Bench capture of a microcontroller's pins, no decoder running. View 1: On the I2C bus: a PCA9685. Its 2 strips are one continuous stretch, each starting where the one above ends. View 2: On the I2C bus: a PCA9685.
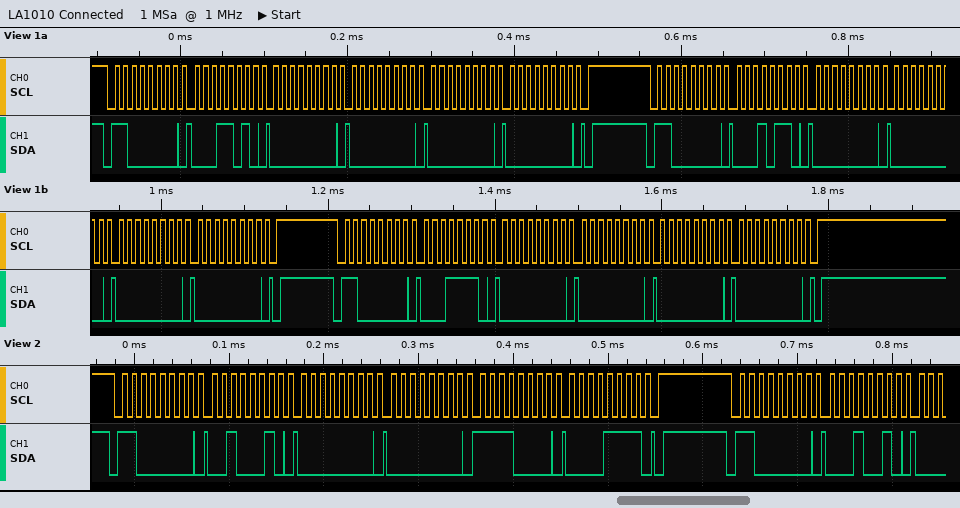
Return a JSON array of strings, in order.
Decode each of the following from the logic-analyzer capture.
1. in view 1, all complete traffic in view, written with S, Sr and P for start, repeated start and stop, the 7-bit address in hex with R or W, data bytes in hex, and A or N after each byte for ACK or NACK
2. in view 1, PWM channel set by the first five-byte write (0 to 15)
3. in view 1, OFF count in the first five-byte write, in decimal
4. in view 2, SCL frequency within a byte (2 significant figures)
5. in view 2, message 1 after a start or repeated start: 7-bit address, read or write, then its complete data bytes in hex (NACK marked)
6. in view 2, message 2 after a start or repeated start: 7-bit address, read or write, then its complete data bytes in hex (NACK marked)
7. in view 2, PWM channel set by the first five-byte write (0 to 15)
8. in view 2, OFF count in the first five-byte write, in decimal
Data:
["S 60W A 1A A 00 A 00 A 00 A 00 A P S 60W A 16 A 00 A 00 A 00 A 00 A P S 60W A 1E A 00 A 00 A 00 A 00 A P", "5", "0", "100 kHz", "0x60 write: 22 00 00 F0 0F", "0x60 write: 12", "7", "4080"]
